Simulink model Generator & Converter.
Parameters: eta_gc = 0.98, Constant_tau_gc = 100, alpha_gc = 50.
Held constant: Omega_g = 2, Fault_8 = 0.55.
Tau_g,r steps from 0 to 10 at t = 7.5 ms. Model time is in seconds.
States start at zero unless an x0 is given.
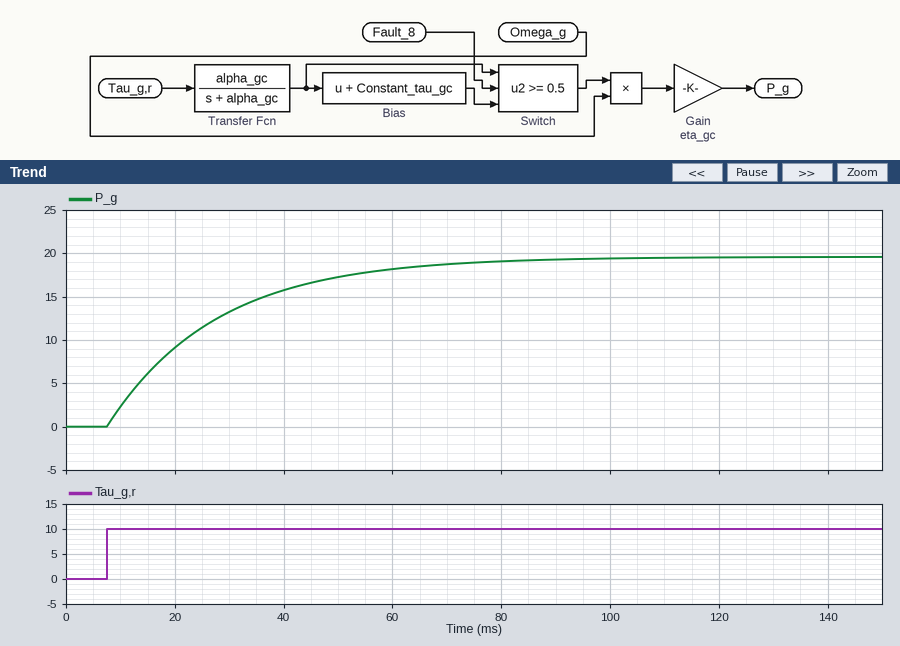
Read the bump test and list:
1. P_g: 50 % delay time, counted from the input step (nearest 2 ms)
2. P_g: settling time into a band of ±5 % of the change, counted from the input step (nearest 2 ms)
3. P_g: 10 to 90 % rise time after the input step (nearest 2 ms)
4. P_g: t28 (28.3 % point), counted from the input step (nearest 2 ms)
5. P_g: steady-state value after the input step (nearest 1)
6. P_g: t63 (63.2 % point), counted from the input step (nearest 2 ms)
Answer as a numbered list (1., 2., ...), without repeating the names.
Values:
1. 14 ms
2. 60 ms
3. 44 ms
4. 6 ms
5. 20
6. 20 ms
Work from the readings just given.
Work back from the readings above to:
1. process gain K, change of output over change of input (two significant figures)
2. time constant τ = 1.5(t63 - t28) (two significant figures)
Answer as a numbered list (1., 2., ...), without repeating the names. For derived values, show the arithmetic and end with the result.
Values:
1. (20 - 0) / 10 = 2.0
2. 1.5 × (20 - 6) = 21 ms
